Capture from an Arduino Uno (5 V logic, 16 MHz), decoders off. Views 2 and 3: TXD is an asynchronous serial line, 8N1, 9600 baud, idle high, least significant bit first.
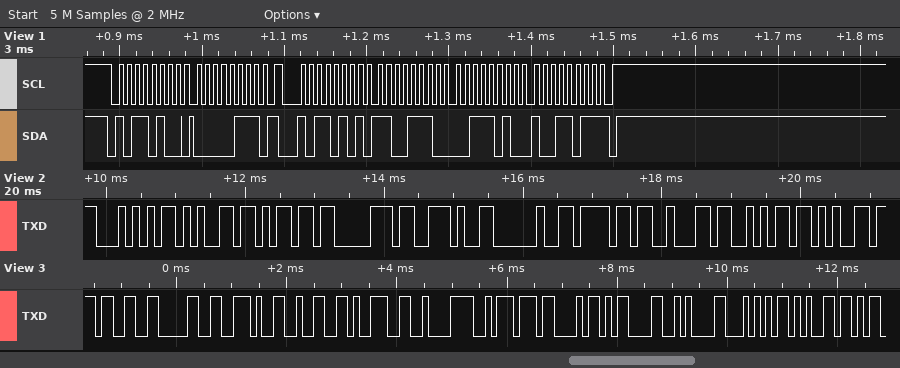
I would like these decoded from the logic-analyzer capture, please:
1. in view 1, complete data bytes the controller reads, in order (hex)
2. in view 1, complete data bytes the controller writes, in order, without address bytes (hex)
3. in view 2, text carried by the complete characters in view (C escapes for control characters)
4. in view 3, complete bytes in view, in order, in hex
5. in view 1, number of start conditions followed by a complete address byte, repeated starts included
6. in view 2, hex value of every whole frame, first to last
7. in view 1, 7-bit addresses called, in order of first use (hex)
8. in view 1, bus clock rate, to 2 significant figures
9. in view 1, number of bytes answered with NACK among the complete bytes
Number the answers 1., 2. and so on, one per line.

1. CE 3A 9B
2. 07
3. "Temp. obje"
4. 0x33 0x30 0x2E 0x32 0x39 0xC2 0xBA 0x43 0x0D 0x0A 0x54 0x65
5. 2
6. 54 65 6D 70 2E 20 6F 62 6A 65
7. 0x5A
8. 100 kHz
9. 1
